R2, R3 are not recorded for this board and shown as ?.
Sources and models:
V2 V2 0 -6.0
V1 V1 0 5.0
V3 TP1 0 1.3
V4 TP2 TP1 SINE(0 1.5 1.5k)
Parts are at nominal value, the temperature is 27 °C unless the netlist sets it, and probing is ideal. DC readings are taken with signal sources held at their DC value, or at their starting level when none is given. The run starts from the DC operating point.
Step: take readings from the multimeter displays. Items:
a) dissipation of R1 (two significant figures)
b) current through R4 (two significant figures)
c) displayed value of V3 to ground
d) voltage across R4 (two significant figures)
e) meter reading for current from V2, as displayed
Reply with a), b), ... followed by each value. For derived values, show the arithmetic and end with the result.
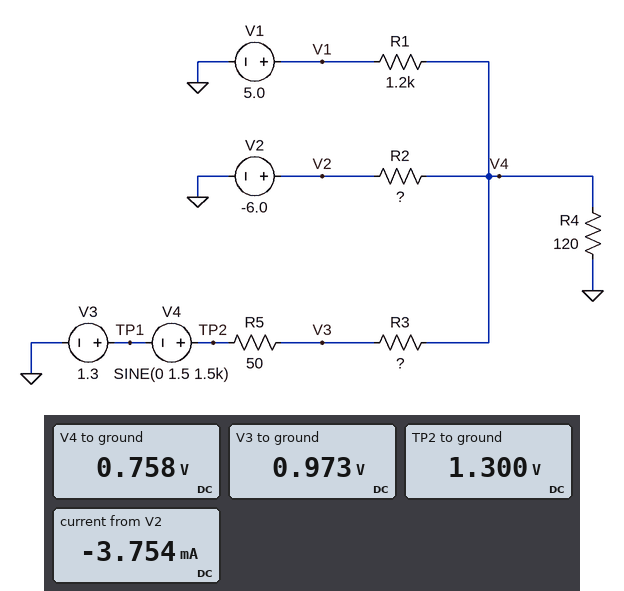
a) (5 V - 758 mV)^2 / 1.2 kΩ = 15 mW
b) (758 mV) / 120 Ω = 6.3 mA
c) 0.973 V
d) 758 mV = 760 mV
e) -3.754 mA
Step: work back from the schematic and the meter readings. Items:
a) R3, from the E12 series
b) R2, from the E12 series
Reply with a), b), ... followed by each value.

a) 33 Ω
b) 1.8 kΩ
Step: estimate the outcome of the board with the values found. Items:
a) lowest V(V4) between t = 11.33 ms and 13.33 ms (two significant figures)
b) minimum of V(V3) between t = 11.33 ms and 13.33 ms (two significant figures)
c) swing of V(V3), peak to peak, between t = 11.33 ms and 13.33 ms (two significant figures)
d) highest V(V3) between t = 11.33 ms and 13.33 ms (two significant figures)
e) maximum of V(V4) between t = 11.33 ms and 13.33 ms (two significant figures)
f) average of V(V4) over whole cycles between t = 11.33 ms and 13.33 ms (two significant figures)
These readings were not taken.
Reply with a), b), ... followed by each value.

a) -72 mV
b) -120 mV
c) 2.2 V
d) 2.1 V
e) 1.6 V
f) 760 mV
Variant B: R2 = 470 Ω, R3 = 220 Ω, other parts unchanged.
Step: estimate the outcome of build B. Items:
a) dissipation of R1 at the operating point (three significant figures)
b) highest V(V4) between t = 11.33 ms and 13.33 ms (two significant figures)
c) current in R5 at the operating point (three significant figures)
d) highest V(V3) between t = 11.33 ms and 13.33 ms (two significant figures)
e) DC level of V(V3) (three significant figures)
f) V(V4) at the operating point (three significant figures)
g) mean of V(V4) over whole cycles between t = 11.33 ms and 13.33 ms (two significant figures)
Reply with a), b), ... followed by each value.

a) 23.0 mW
b) 120 mV
c) 5.75 mA
d) 2.3 V
e) 1.01 V
f) -252 mV
g) -250 mV
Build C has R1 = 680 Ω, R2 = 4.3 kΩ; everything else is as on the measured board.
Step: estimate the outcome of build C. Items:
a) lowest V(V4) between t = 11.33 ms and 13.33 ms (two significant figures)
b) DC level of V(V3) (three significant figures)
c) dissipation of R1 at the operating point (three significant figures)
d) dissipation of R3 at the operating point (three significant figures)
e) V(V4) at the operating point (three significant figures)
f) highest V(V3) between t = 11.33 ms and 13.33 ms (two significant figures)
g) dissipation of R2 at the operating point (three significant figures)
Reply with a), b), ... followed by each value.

a) 160 mV
b) 1.11 V
c) 23.8 mW
d) 494 µW
e) 979 mV
f) 2.2 V
g) 11.3 mW
